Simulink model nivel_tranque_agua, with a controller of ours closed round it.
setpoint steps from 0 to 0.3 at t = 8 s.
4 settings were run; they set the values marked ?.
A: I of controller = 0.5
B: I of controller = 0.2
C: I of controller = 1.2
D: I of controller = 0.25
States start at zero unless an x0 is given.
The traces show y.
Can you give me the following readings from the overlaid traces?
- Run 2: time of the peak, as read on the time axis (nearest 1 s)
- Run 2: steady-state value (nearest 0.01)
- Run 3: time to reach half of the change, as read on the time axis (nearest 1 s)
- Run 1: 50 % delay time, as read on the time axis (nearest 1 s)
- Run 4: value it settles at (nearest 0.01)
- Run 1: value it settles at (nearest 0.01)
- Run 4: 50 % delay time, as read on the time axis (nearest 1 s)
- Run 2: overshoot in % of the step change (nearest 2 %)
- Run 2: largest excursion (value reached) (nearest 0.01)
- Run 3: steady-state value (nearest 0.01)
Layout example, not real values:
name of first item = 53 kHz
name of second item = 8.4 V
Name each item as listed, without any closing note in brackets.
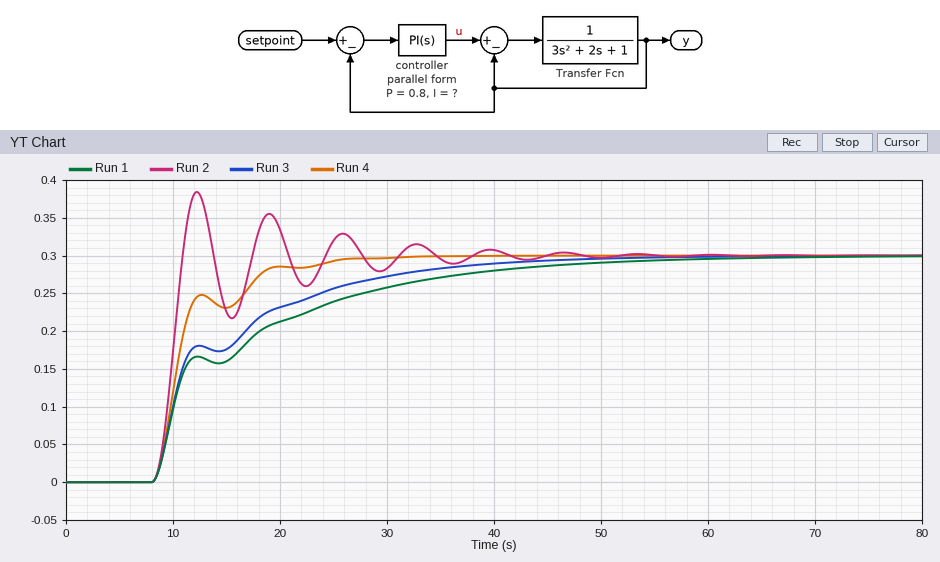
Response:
Run 2: time of the peak, as read on the time axis = 12 s
Run 2: steady-state value = 0.30
Run 3: time to reach half of the change, as read on the time axis = 11 s
Run 1: 50 % delay time, as read on the time axis = 11 s
Run 4: value it settles at = 0.30
Run 1: value it settles at = 0.30
Run 4: 50 % delay time, as read on the time axis = 10 s
Run 2: overshoot in % of the step change = 28 %
Run 2: largest excursion (value reached) = 0.38
Run 3: steady-state value = 0.30
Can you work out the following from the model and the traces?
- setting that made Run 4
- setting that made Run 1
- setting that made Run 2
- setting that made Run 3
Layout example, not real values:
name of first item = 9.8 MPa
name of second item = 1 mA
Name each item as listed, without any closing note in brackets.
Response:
setting that made Run 4 = A
setting that made Run 1 = B
setting that made Run 2 = C
setting that made Run 3 = D
